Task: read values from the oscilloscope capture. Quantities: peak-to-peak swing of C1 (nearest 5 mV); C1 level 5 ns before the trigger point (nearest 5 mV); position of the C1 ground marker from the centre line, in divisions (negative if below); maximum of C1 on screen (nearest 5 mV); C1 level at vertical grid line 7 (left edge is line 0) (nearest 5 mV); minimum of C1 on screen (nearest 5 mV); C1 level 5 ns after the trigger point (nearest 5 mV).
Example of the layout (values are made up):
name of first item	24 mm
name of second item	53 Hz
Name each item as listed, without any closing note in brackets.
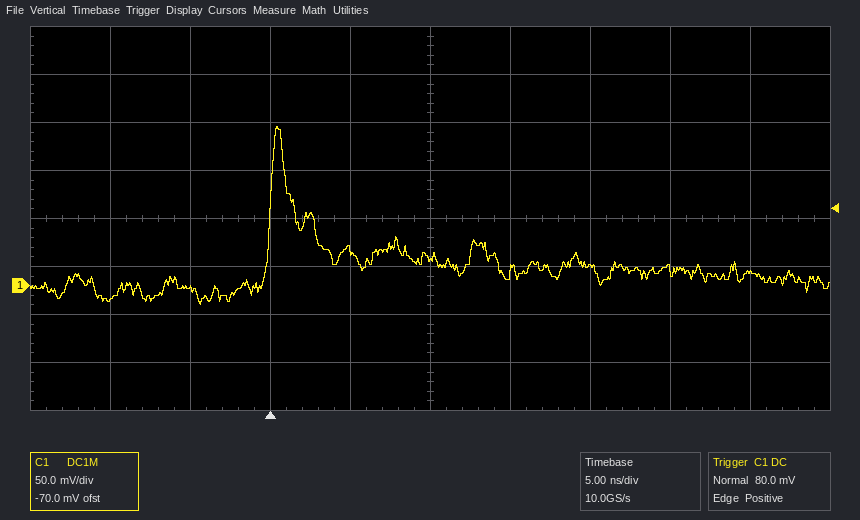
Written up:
peak-to-peak swing of C1	185 mV
C1 level 5 ns before the trigger point	-5 mV
position of the C1 ground marker from the centre line, in divisions	-1.4 div
maximum of C1 on screen	165 mV
C1 level at vertical grid line 7 (left edge is line 0)	20 mV
minimum of C1 on screen	-20 mV
C1 level 5 ns after the trigger point	35 mV
